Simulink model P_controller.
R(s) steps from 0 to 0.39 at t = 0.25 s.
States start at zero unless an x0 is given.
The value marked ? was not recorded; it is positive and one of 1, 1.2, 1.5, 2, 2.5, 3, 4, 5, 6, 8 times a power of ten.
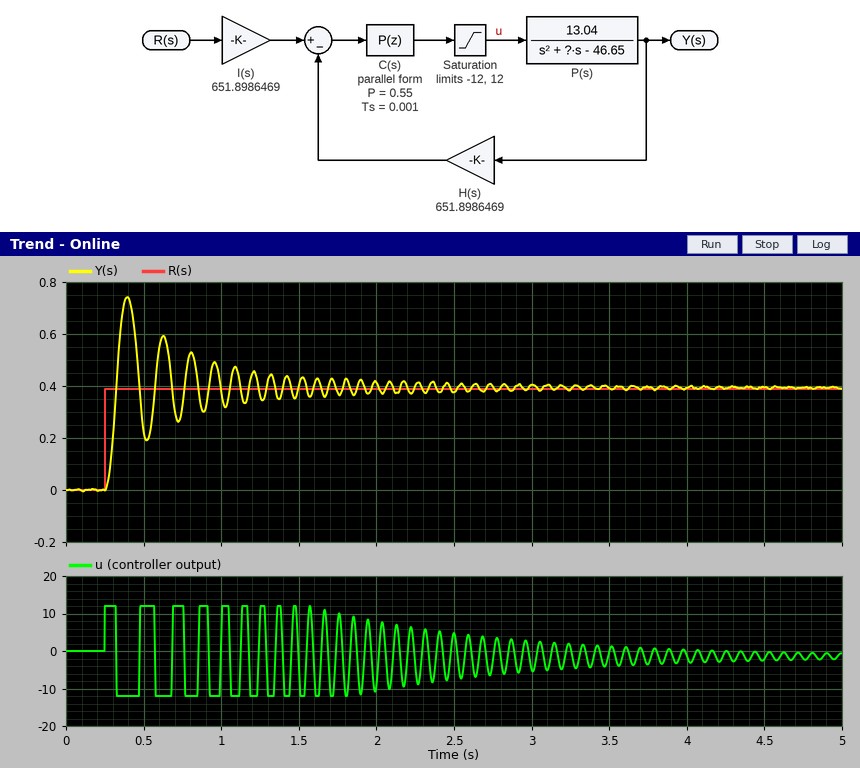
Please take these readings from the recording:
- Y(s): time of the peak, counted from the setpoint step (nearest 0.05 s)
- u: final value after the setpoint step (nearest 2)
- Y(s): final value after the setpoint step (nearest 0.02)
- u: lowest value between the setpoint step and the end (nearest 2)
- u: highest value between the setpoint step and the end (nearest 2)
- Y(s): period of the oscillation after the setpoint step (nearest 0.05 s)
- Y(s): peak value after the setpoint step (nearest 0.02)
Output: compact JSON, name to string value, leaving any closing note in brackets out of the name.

{"Y(s): time of the peak, counted from the setpoint step": "0.15 s", "u: final value after the setpoint step": "-2", "Y(s): final value after the setpoint step": "0.40", "u: lowest value between the setpoint step and the end": "-12", "u: highest value between the setpoint step and the end": "12", "Y(s): period of the oscillation after the setpoint step": "0.25 s", "Y(s): peak value after the setpoint step": "0.74"}
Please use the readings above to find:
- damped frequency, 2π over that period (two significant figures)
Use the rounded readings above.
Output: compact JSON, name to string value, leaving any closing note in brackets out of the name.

{"damped frequency, 2π over that period": "25 rad/s"}
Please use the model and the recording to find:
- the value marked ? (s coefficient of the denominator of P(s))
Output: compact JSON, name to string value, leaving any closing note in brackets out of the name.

{"the value marked ? (s coefficient of the denominator of P(s))": "4"}
